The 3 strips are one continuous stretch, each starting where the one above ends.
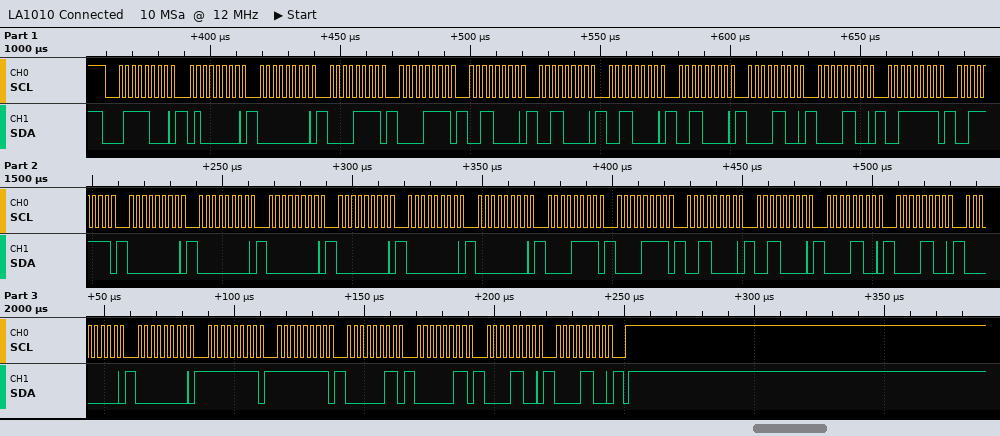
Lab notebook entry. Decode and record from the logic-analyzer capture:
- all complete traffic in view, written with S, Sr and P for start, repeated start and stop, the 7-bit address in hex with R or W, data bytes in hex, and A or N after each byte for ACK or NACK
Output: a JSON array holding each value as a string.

["S 3CW A 40 A 00 A 0F A 0F A 30 A 30 A 30 A 30 A 0C A 0C A 3F A 3F A 00 A 00 A 00 A 00 A 00 A 00 A 0F A 0F A 30 A 30 A 0C A 0C A 00 A 00 A FF A FF A 03 A 03 A 0C A 0C A P"]
